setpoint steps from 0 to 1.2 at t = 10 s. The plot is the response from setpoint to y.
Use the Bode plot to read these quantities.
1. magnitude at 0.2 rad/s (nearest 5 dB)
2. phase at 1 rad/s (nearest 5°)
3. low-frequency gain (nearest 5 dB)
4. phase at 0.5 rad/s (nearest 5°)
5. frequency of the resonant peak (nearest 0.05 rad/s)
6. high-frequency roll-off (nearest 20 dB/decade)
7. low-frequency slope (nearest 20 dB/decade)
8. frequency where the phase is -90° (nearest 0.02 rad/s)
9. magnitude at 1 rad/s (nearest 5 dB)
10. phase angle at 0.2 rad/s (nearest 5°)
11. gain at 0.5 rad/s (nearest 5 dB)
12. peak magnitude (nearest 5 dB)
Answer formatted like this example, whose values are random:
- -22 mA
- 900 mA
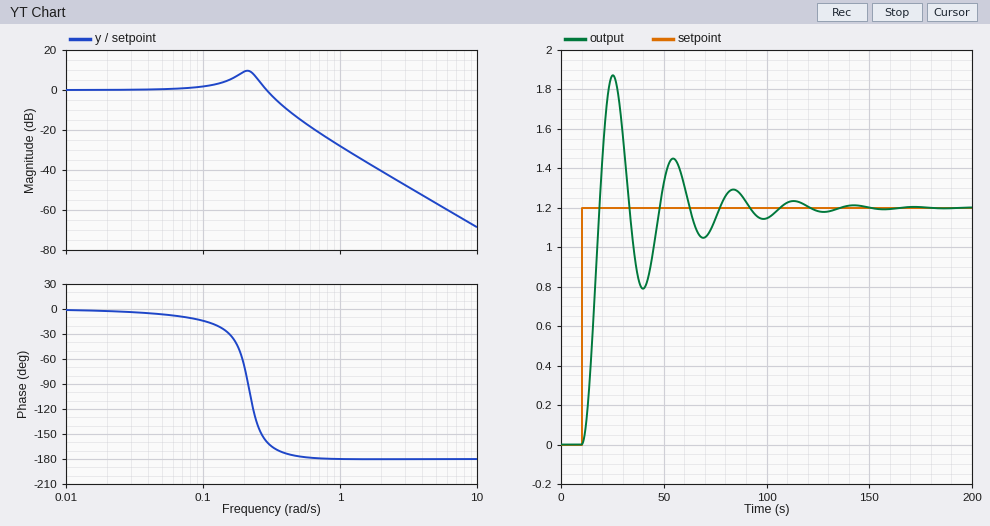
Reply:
- 10 dB
- -180°
- 0 dB
- -175°
- 0.20 rad/s
- -40 dB/decade
- 0 dB/decade
- 0.22 rad/s
- -30 dB
- -70°
- -15 dB
- 10 dB
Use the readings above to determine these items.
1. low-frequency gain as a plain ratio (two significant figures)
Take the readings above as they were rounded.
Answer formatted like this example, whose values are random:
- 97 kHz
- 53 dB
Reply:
- 1.0
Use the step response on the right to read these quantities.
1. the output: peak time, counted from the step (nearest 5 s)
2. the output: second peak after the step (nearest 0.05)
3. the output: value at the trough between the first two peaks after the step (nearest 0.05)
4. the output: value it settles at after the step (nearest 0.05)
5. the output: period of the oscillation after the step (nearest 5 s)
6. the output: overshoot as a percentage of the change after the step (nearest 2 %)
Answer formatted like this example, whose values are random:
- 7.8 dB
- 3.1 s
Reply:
- 15 s
- 1.45
- 0.80
- 1.20
- 30 s
- 56 %
